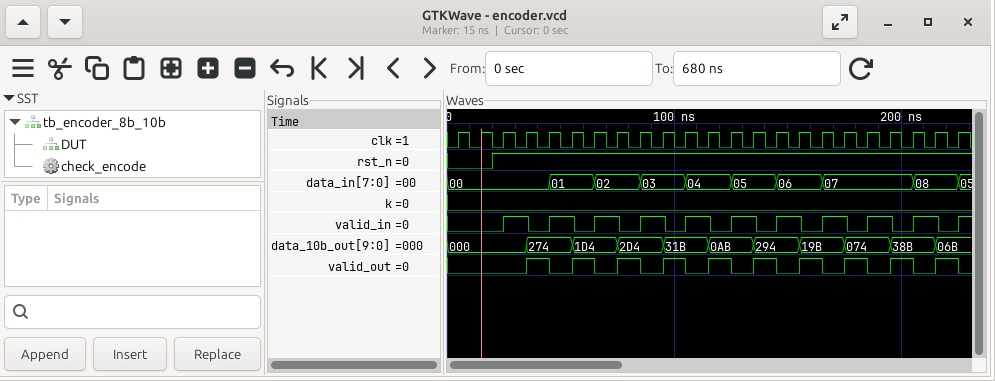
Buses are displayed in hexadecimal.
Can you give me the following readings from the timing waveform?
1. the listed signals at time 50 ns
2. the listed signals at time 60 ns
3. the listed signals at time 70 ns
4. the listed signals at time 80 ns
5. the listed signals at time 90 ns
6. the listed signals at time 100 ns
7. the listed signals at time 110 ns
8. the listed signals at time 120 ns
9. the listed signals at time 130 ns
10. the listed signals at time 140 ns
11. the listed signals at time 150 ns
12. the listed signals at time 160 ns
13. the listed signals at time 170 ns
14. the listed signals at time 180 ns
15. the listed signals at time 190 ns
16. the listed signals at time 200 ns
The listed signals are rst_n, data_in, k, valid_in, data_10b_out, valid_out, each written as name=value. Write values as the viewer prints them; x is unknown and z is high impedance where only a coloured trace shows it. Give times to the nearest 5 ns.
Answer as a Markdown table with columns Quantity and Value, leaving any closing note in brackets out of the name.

| Quantity | Value |
|---|---|
| the listed signals at time 50 ns | rst_n=1, data_in=01, k=0, valid_in=1, data_10b_out=274, valid_out=0 |
| the listed signals at time 60 ns | rst_n=1, data_in=01, k=0, valid_in=0, data_10b_out=1D4, valid_out=1 |
| the listed signals at time 70 ns | rst_n=1, data_in=02, k=0, valid_in=1, data_10b_out=1D4, valid_out=0 |
| the listed signals at time 80 ns | rst_n=1, data_in=02, k=0, valid_in=0, data_10b_out=2D4, valid_out=1 |
| the listed signals at time 90 ns | rst_n=1, data_in=03, k=0, valid_in=1, data_10b_out=2D4, valid_out=0 |
| the listed signals at time 100 ns | rst_n=1, data_in=03, k=0, valid_in=0, data_10b_out=31B, valid_out=1 |
| the listed signals at time 110 ns | rst_n=1, data_in=04, k=0, valid_in=1, data_10b_out=31B, valid_out=0 |
| the listed signals at time 120 ns | rst_n=1, data_in=04, k=0, valid_in=0, data_10b_out=0AB, valid_out=1 |
| the listed signals at time 130 ns | rst_n=1, data_in=05, k=0, valid_in=1, data_10b_out=0AB, valid_out=0 |
| the listed signals at time 140 ns | rst_n=1, data_in=05, k=0, valid_in=0, data_10b_out=294, valid_out=1 |
| the listed signals at time 150 ns | rst_n=1, data_in=06, k=0, valid_in=1, data_10b_out=294, valid_out=0 |
| the listed signals at time 160 ns | rst_n=1, data_in=06, k=0, valid_in=0, data_10b_out=19B, valid_out=1 |
| the listed signals at time 170 ns | rst_n=1, data_in=07, k=0, valid_in=1, data_10b_out=19B, valid_out=0 |
| the listed signals at time 180 ns | rst_n=1, data_in=07, k=0, valid_in=0, data_10b_out=074, valid_out=1 |
| the listed signals at time 190 ns | rst_n=1, data_in=07, k=0, valid_in=1, data_10b_out=074, valid_out=0 |
| the listed signals at time 200 ns | rst_n=1, data_in=07, k=0, valid_in=0, data_10b_out=38B, valid_out=1 |
